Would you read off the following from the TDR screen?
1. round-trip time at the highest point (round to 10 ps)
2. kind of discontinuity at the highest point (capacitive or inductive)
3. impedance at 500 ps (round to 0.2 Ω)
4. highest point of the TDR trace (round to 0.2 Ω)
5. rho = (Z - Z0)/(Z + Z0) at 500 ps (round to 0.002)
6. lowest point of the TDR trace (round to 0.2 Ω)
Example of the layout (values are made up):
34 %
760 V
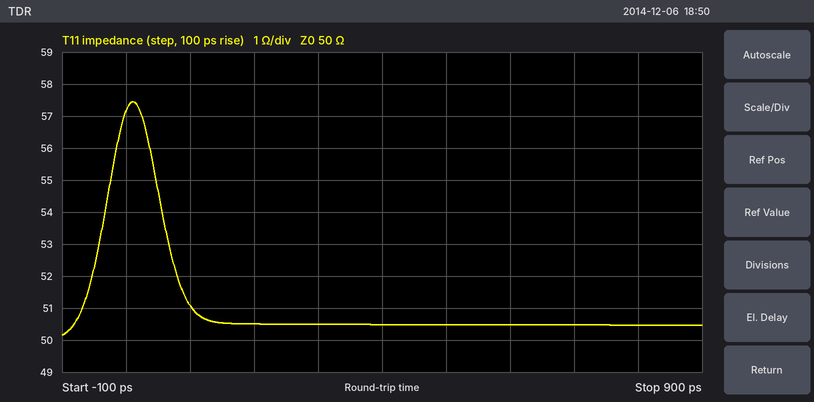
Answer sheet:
10 ps
inductive
50.4 Ω
57.4 Ω
+0.004
50.2 Ω
